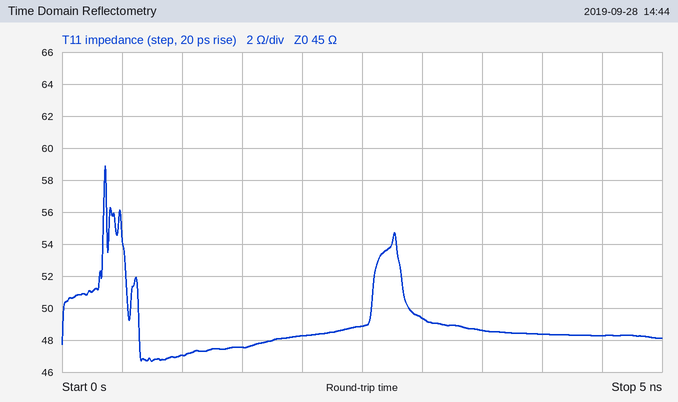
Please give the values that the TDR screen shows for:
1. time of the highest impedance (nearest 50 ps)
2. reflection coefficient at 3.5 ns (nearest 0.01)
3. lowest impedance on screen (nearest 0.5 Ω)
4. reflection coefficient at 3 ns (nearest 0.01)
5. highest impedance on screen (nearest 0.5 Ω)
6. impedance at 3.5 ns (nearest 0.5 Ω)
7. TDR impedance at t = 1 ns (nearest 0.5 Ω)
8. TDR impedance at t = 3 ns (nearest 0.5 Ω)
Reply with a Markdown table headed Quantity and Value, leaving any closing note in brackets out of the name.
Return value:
| Quantity | Value |
|---|---|
| time of the highest impedance | 350 ps |
| reflection coefficient at 3.5 ns | +0.04 |
| lowest impedance on screen | 46.5 Ω |
| reflection coefficient at 3 ns | +0.05 |
| highest impedance on screen | 59.0 Ω |
| impedance at 3.5 ns | 48.5 Ω |
| TDR impedance at t = 1 ns | 47.0 Ω |
| TDR impedance at t = 3 ns | 49.5 Ω |
